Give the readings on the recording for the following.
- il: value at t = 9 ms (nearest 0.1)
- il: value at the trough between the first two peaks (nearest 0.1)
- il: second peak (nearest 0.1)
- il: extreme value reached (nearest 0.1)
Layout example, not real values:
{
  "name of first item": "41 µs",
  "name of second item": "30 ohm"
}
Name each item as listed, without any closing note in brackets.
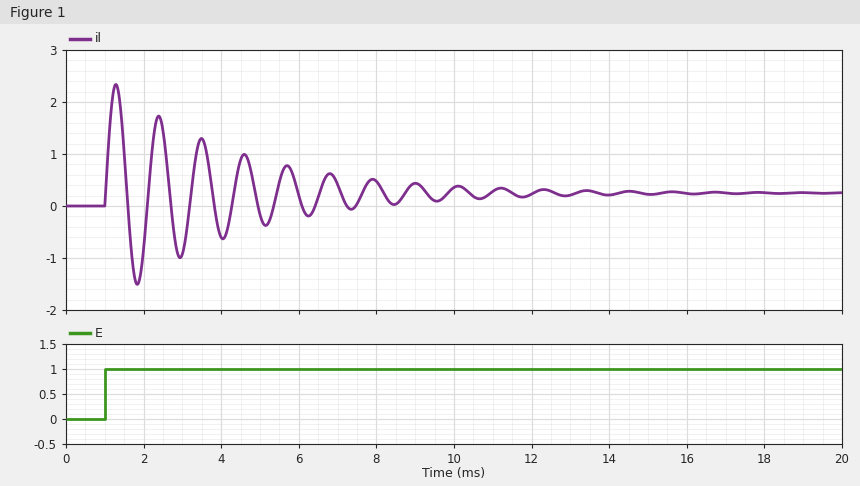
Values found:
{
  "il: value at t = 9 ms": "0.4",
  "il: value at the trough between the first two peaks": "-1.5",
  "il: second peak": "1.7",
  "il: extreme value reached": "2.3"
}
